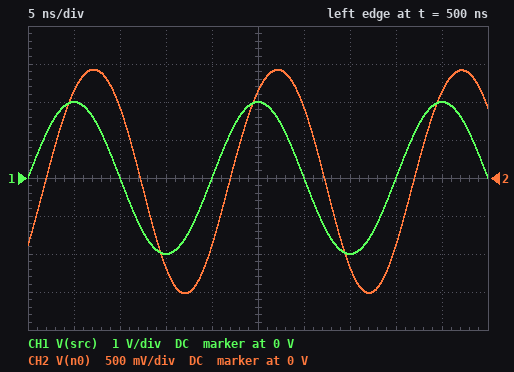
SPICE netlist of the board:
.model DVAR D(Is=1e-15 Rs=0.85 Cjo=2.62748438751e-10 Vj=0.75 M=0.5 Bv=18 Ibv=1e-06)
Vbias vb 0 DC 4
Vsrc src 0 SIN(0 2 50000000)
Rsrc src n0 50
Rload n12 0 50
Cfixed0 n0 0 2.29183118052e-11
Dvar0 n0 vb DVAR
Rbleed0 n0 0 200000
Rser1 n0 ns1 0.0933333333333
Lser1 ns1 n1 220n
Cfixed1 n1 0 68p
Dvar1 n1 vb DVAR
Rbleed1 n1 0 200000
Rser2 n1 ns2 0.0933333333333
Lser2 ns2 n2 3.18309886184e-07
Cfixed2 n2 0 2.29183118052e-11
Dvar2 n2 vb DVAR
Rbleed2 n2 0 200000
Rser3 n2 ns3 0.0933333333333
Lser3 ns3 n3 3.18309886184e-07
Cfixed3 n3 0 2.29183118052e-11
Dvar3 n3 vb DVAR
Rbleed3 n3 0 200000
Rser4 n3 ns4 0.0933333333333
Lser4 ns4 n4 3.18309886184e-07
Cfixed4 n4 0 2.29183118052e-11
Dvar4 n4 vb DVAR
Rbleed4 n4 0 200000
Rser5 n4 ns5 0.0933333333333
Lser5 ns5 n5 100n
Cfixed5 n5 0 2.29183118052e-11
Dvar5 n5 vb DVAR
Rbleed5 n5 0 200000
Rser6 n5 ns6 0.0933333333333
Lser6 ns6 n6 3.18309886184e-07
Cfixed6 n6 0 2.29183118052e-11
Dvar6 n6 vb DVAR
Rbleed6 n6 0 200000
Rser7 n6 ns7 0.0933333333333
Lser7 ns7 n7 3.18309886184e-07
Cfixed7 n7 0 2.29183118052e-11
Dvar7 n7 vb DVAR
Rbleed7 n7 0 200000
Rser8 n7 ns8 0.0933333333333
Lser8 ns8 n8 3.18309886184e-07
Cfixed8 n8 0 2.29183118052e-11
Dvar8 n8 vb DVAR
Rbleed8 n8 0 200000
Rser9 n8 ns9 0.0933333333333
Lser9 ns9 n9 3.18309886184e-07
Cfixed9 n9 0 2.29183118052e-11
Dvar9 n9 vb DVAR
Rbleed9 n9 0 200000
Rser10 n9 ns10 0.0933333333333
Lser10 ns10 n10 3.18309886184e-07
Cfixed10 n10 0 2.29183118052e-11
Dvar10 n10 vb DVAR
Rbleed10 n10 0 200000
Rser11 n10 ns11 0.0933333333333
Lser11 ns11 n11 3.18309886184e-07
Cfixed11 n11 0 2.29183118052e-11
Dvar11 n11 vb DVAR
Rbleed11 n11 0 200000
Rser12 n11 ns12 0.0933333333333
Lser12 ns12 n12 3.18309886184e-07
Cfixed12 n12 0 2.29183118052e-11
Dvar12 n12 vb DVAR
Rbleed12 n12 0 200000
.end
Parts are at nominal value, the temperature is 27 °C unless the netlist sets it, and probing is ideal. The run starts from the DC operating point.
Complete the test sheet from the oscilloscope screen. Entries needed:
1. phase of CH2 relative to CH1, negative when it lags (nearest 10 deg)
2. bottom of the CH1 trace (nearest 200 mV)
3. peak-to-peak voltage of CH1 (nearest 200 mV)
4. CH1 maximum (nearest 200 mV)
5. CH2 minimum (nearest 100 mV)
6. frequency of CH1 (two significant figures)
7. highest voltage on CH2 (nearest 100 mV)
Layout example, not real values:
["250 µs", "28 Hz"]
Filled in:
["-40 deg", "-2.0 V", "4.0 V", "2.0 V", "-1.5 V", "50 MHz", "1.4 V"]
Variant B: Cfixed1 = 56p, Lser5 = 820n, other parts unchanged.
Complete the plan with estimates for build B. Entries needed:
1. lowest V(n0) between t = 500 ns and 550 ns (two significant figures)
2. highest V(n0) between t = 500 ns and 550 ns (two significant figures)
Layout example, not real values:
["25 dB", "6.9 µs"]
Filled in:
["-1.6 V", "1.5 V"]
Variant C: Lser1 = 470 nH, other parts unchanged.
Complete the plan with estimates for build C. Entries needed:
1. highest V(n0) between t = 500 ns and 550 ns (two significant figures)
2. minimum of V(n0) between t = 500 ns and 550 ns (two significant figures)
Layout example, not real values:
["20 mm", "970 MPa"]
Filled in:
["1.0 V", "-1.1 V"]
